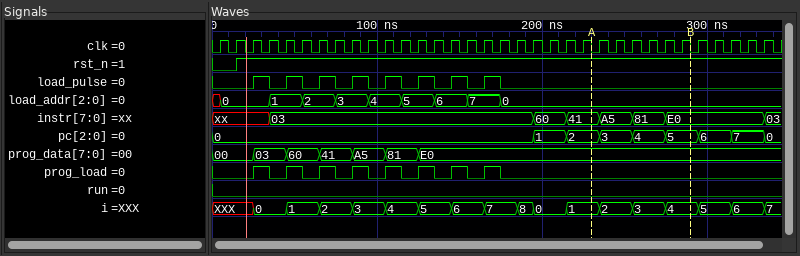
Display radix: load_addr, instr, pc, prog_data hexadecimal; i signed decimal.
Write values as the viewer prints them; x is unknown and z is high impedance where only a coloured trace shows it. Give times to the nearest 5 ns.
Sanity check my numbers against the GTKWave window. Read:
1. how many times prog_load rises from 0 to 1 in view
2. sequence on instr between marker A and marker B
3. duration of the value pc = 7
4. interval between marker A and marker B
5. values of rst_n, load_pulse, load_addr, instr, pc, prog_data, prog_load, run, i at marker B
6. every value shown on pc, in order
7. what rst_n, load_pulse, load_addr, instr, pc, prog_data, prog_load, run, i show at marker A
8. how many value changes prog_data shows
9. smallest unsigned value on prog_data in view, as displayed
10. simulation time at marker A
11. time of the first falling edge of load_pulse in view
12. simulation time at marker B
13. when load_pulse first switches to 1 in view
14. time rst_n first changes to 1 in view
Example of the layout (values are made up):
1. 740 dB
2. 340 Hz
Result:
1. 8
2. 41, A5, 81, E0
3. 20 ns
4. 60 ns
5. rst_n=1, load_pulse=0, load_addr=0, instr=E0, pc=5, prog_data=E0, prog_load=0, run=0, i=4
6. 0, 1, 2, 3, 4, 5, 6, 7, 0
7. rst_n=1, load_pulse=0, load_addr=0, instr=41, pc=2, prog_data=E0, prog_load=0, run=0, i=1
8. 6
9. 00
10. 230 ns
11. 35 ns
12. 290 ns
13. 25 ns
14. 15 ns
